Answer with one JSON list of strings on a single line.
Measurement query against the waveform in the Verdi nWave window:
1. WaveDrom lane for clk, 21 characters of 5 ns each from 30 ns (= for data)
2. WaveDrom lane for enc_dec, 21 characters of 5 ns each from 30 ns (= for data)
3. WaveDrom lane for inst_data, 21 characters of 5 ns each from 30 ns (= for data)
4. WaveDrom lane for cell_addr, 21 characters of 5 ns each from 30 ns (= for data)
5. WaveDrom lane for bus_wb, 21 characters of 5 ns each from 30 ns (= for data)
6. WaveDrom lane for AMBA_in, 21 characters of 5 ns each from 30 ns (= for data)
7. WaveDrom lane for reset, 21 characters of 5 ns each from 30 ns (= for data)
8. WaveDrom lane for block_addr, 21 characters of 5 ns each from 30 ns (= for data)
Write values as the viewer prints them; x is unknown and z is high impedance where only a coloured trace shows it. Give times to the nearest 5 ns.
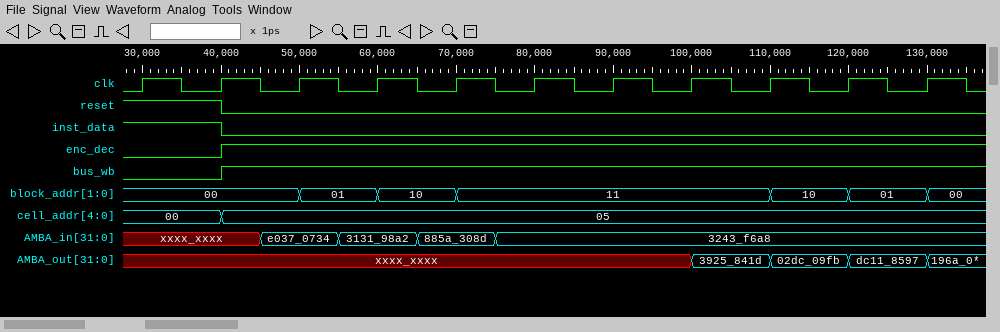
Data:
["{name: 'clk', wave: '101010101010101010101'}", "{name: 'enc_dec', wave: '0.1..................'}", "{name: 'inst_data', wave: '1.0..................'}", "{name: 'cell_addr', wave: '=.=..................', data: '00 05'}", "{name: 'bus_wb', wave: '0.1..................'}", "{name: 'AMBA_in', wave: 'x..=.=.=.=...........', data: 'e037_0734 3131_98a2 885a_308d 3243_f6a8'}", "{name: 'reset', wave: '1.0..................'}", "{name: 'block_addr', wave: '=...=.=.=.......=.=.=', data: '00 01 10 11 10 01 00'}"]
